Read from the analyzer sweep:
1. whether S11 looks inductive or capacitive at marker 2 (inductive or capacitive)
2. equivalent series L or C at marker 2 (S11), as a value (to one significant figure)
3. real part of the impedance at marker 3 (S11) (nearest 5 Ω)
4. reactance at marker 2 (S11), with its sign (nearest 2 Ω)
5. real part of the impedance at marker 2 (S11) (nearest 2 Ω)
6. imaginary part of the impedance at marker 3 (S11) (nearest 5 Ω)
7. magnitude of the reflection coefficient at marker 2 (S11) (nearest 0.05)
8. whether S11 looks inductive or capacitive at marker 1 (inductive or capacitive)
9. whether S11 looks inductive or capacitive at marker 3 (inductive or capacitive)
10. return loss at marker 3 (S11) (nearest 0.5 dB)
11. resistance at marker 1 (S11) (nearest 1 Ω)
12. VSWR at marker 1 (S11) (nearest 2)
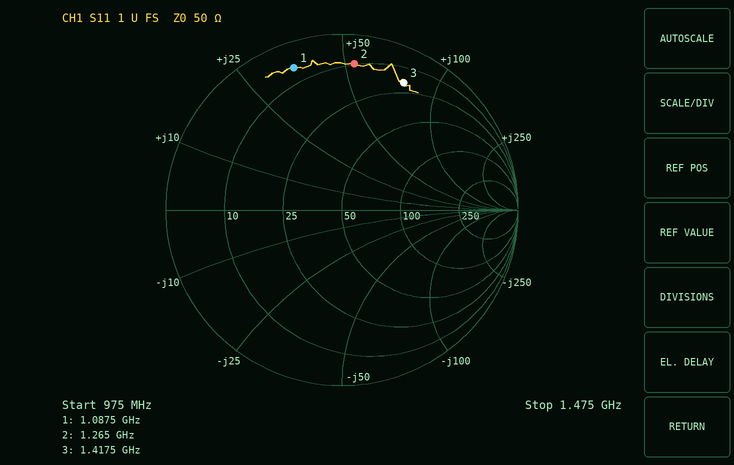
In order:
inductive
7 nH
20 Ω
+54 Ω
10 Ω
+75 Ω
0.85
inductive
inductive
2.0 dB
6 Ω
12
